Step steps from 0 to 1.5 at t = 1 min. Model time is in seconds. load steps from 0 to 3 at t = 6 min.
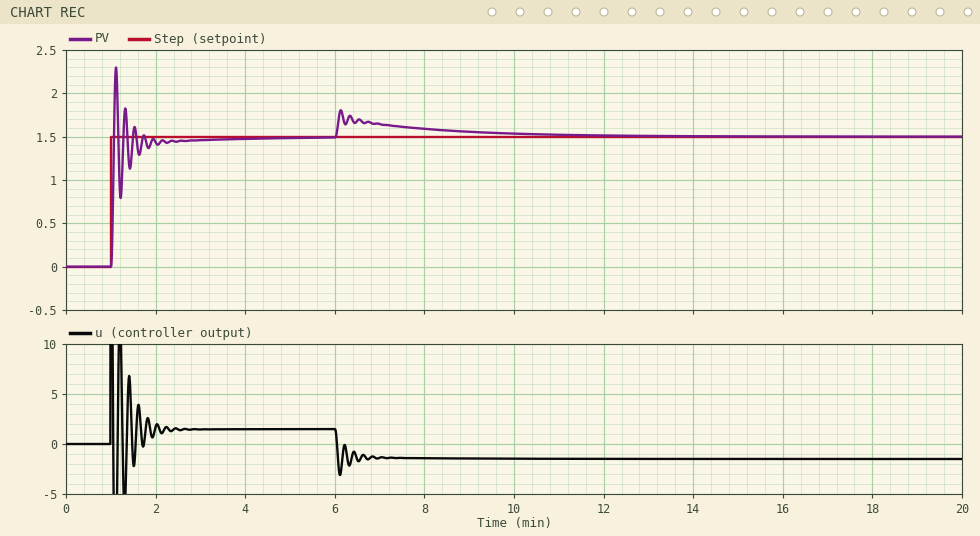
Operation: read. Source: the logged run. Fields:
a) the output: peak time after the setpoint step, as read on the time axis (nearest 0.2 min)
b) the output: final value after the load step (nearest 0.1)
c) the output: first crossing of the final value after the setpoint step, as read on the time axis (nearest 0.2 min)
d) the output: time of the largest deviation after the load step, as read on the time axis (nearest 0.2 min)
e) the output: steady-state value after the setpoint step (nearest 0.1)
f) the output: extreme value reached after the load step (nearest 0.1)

1.2 min
1.5
1.0 min
6.2 min
1.5
1.8
